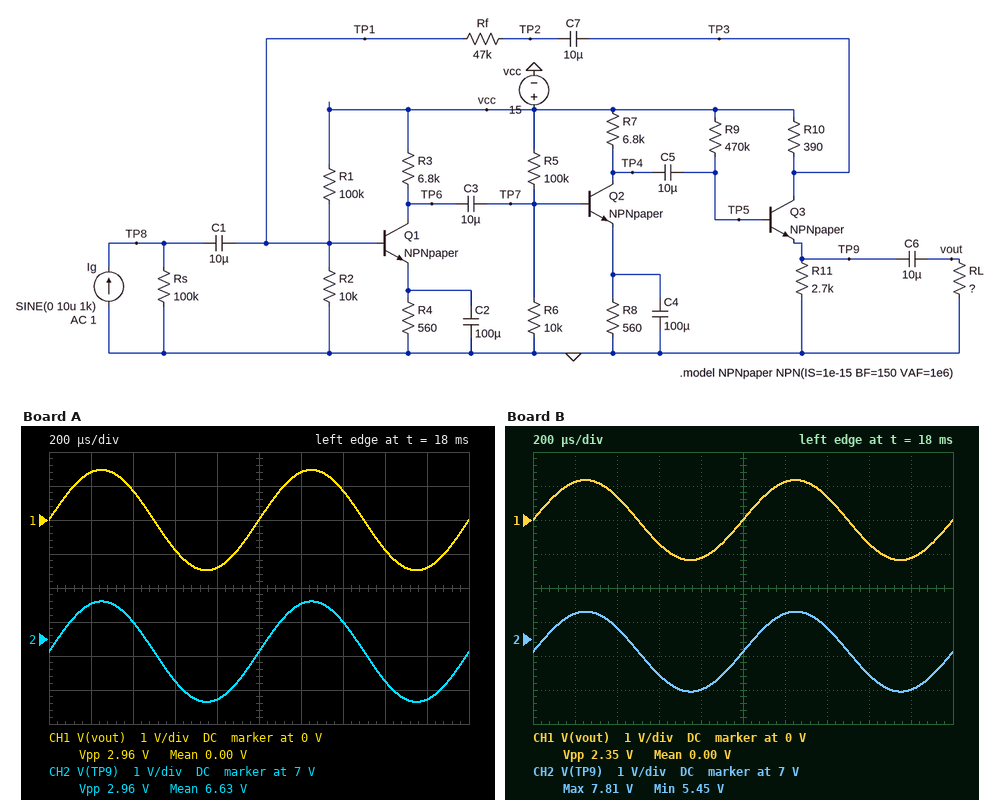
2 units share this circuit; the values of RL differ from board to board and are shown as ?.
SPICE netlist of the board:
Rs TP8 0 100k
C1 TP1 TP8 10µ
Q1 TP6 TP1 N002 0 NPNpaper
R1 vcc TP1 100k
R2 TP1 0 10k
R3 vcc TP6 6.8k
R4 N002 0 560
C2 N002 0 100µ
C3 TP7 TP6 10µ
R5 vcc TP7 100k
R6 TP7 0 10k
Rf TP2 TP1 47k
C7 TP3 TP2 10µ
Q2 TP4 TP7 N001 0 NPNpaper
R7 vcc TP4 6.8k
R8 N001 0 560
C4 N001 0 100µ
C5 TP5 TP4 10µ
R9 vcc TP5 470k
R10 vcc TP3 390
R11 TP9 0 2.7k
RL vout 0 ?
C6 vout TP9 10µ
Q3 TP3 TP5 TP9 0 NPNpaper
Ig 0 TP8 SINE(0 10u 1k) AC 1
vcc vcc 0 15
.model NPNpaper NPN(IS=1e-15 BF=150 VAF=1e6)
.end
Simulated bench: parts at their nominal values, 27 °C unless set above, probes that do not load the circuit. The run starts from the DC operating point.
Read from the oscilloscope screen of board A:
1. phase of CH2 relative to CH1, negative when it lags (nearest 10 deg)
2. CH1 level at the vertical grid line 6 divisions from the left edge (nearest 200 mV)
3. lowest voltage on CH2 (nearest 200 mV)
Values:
0 deg
1.4 V
5.2 V
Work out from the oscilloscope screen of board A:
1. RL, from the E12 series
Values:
2.2 kΩ
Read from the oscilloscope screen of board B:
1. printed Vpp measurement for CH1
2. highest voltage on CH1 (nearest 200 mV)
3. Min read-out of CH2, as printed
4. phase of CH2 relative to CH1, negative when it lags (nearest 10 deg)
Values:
2.35 V
1.2 V
5.45 V
0 deg
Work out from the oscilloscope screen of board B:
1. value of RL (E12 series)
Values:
1.5 kΩ
